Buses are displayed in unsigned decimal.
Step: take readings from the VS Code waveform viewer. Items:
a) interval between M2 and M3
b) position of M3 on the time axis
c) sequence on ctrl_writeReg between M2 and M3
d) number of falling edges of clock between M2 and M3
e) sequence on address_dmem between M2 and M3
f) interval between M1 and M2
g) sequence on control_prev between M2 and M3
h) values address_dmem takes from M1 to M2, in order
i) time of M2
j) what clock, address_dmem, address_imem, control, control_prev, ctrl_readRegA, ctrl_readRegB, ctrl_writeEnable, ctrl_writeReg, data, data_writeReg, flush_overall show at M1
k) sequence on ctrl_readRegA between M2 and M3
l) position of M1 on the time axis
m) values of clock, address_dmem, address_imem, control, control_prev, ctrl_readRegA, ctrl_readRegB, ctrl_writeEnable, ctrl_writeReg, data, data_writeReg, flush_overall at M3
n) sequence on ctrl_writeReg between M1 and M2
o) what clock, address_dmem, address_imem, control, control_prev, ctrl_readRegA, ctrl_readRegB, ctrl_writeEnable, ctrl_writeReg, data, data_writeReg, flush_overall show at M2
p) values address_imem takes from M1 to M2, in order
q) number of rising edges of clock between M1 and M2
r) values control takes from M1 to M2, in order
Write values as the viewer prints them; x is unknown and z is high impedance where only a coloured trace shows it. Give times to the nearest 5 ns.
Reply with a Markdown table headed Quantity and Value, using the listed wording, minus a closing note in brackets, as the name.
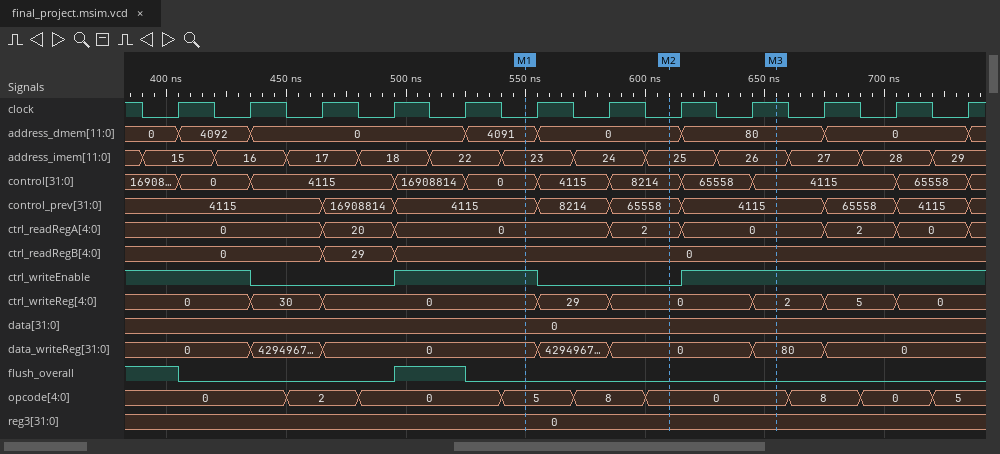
| Quantity | Value |
|---|---|
| interval between M2 and M3 | 45 ns |
| position of M3 on the time axis | 655 ns |
| sequence on ctrl_writeReg between M2 and M3 | 0, 2 |
| number of falling edges of clock between M2 and M3 | 1 |
| sequence on address_dmem between M2 and M3 | 0, 80 |
| interval between M1 and M2 | 60 ns |
| sequence on control_prev between M2 and M3 | 65558, 4115 |
| values address_dmem takes from M1 to M2, in order | 4091, 0 |
| time of M2 | 610 ns |
| what clock, address_dmem, address_imem, control, control_prev, ctrl_readRegA, ctrl_readRegB, ctrl_writeEnable, ctrl_writeReg, data, data_writeReg, flush_overall show at M1 | clock=0, address_dmem=4091, address_imem=23, control=0, control_prev=4115, ctrl_readRegA=0, ctrl_readRegB=0, ctrl_writeEnable=1, ctrl_writeReg=0, data=0, data_writeReg=0, flush_overall=0 |
| sequence on ctrl_readRegA between M2 and M3 | 2, 0 |
| position of M1 on the time axis | 550 ns |
| values of clock, address_dmem, address_imem, control, control_prev, ctrl_readRegA, ctrl_readRegB, ctrl_writeEnable, ctrl_writeReg, data, data_writeReg, flush_overall at M3 | clock=1, address_dmem=80, address_imem=26, control=4115, control_prev=4115, ctrl_readRegA=0, ctrl_readRegB=0, ctrl_writeEnable=1, ctrl_writeReg=2, data=0, data_writeReg=80, flush_overall=0 |
| sequence on ctrl_writeReg between M1 and M2 | 0, 29, 0 |
| what clock, address_dmem, address_imem, control, control_prev, ctrl_readRegA, ctrl_readRegB, ctrl_writeEnable, ctrl_writeReg, data, data_writeReg, flush_overall show at M2 | clock=0, address_dmem=0, address_imem=25, control=8214, control_prev=65558, ctrl_readRegA=2, ctrl_readRegB=0, ctrl_writeEnable=0, ctrl_writeReg=0, data=0, data_writeReg=0, flush_overall=0 |
| values address_imem takes from M1 to M2, in order | 23, 24, 25 |
| number of rising edges of clock between M1 and M2 | 2 |
| values control takes from M1 to M2, in order | 0, 4115, 8214 |
